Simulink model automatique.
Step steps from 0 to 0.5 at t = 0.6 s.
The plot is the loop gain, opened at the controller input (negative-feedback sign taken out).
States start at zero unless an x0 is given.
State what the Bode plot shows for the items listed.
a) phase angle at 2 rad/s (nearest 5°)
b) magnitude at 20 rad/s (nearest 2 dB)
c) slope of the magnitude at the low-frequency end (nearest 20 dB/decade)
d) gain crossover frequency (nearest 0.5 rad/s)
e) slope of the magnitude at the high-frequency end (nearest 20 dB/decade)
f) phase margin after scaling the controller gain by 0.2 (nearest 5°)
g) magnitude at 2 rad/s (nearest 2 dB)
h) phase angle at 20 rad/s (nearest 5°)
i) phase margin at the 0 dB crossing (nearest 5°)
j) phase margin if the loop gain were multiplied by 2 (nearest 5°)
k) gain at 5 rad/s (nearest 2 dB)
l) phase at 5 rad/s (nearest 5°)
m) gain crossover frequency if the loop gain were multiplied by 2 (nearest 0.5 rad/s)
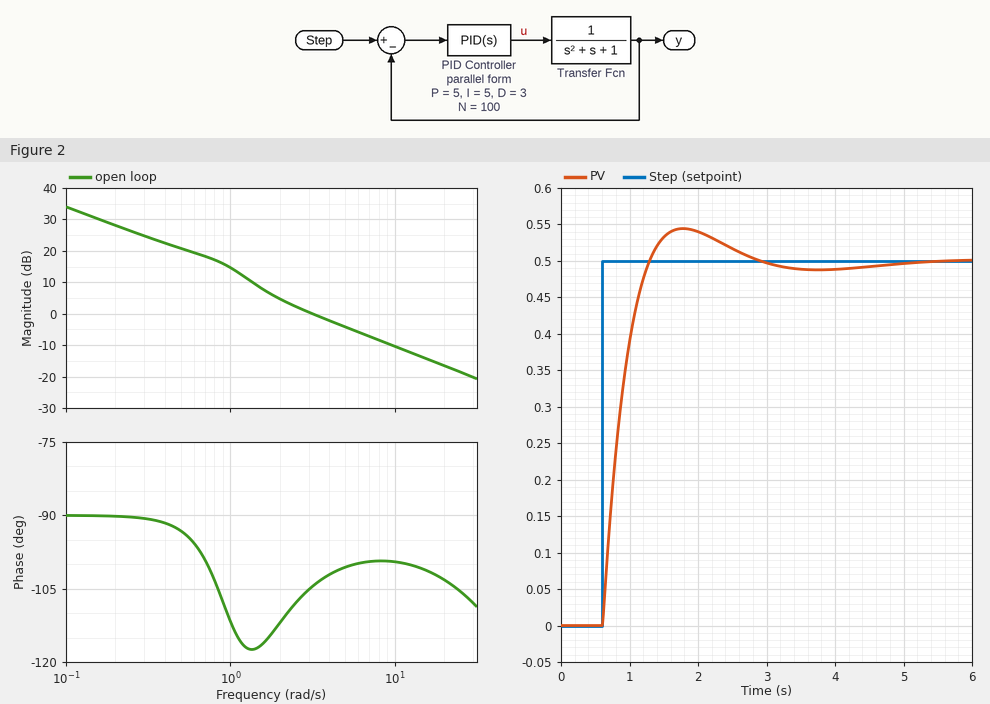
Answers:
-110°
-16 dB
-20 dB/decade
3.0 rad/s
-20 dB/decade
65°
4 dB
-105°
75°
80°
-4 dB
-100°
6.0 rad/s
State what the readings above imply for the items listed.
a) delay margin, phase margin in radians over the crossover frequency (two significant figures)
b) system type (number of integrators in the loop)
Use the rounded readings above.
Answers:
0.44 s
1
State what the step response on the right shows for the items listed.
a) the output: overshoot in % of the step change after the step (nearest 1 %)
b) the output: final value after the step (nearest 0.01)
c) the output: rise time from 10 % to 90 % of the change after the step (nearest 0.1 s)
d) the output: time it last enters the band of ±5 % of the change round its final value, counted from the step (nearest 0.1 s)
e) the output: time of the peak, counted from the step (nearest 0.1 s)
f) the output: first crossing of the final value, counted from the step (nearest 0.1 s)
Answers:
9 %
0.50
0.5 s
1.7 s
1.2 s
0.7 s
